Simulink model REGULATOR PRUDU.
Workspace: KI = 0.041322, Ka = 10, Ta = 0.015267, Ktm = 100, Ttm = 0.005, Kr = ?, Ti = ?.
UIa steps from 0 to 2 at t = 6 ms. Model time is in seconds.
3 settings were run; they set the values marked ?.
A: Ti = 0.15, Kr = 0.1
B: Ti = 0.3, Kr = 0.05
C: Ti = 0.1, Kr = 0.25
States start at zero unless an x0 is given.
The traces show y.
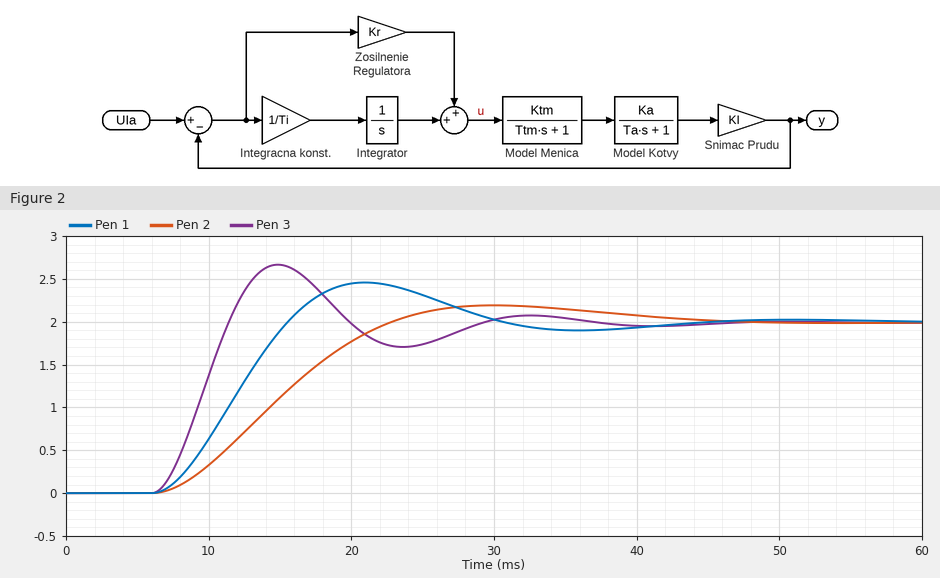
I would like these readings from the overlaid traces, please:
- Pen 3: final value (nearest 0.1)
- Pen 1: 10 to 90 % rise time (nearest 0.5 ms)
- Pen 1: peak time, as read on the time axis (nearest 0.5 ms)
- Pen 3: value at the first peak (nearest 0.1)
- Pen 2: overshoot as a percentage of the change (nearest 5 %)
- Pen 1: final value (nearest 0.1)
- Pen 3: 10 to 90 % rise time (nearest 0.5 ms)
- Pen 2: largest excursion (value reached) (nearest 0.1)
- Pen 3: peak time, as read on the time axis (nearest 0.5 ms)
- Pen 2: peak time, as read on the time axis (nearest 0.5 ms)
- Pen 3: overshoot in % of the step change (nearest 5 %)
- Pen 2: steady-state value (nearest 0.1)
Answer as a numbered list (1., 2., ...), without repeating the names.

1. 2.0
2. 6.5 ms
3. 21.0 ms
4. 2.7
5. 10 %
6. 2.0
7. 3.5 ms
8. 2.2
9. 15.0 ms
10. 30.0 ms
11. 35 %
12. 2.0
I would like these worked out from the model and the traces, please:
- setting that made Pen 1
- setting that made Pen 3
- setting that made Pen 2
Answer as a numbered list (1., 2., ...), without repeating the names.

1. A
2. C
3. B
